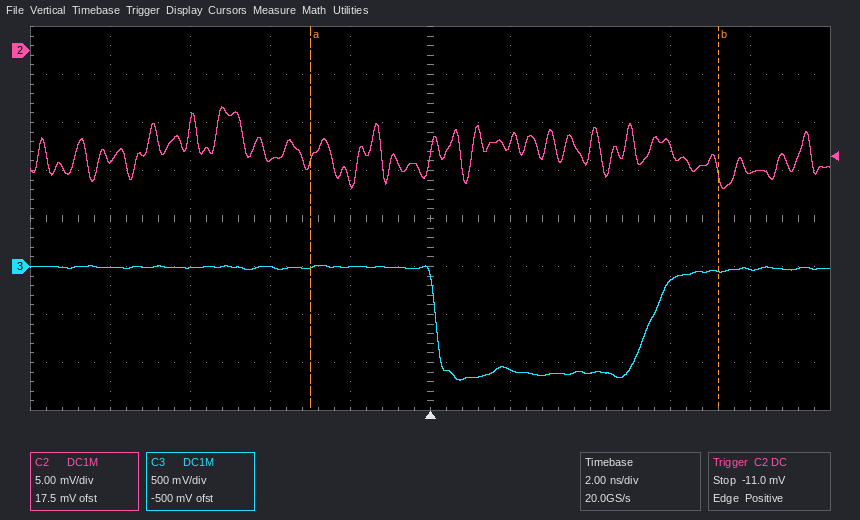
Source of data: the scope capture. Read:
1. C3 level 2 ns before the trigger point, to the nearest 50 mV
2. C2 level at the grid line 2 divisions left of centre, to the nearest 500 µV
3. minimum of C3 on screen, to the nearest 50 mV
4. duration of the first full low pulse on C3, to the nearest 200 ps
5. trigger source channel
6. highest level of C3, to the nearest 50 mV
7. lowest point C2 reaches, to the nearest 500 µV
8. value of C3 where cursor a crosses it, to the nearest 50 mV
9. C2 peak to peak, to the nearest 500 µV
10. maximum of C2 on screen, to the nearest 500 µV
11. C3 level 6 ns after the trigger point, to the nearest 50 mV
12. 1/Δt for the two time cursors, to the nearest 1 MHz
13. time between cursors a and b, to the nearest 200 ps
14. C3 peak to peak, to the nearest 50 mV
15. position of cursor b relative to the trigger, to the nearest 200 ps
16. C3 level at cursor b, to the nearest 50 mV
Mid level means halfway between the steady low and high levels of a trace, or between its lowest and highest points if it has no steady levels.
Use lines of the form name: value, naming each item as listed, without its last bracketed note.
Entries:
C3 level 2 ns before the trigger point, to the nearest 50 mV: 0 mV
C2 level at the grid line 2 divisions left of centre, to the nearest 500 µV: -11.5 mV
minimum of C3 on screen, to the nearest 50 mV: -1.20 V
duration of the first full low pulse on C3, to the nearest 200 ps: 5.4 ns
trigger source channel: C2
highest level of C3, to the nearest 50 mV: 0 mV
lowest point C2 reaches, to the nearest 500 µV: -14.5 mV
value of C3 where cursor a crosses it, to the nearest 50 mV: 0 mV
C2 peak to peak, to the nearest 500 µV: 8.5 mV
maximum of C2 on screen, to the nearest 500 µV: -6.0 mV
C3 level 6 ns after the trigger point, to the nearest 50 mV: -150 mV
1/Δt for the two time cursors, to the nearest 1 MHz: 98 MHz
time between cursors a and b, to the nearest 200 ps: 10.2 ns
C3 peak to peak, to the nearest 50 mV: 1.20 V
position of cursor b relative to the trigger, to the nearest 200 ps: +7.2 ns
C3 level at cursor b, to the nearest 50 mV: -50 mV
